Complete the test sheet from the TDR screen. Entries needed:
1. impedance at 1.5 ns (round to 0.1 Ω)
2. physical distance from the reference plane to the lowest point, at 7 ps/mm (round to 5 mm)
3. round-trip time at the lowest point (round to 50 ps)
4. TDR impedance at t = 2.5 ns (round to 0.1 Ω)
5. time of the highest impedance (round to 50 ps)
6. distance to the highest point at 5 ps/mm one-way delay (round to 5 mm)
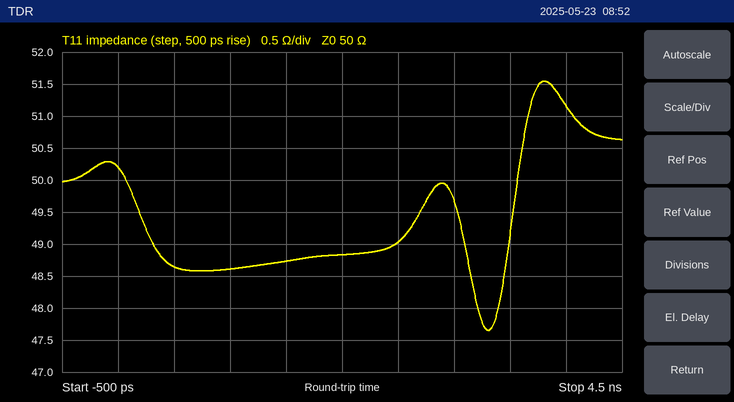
48.7 Ω
235 mm
3.30 ns
49.0 Ω
3.80 ns
380 mm
